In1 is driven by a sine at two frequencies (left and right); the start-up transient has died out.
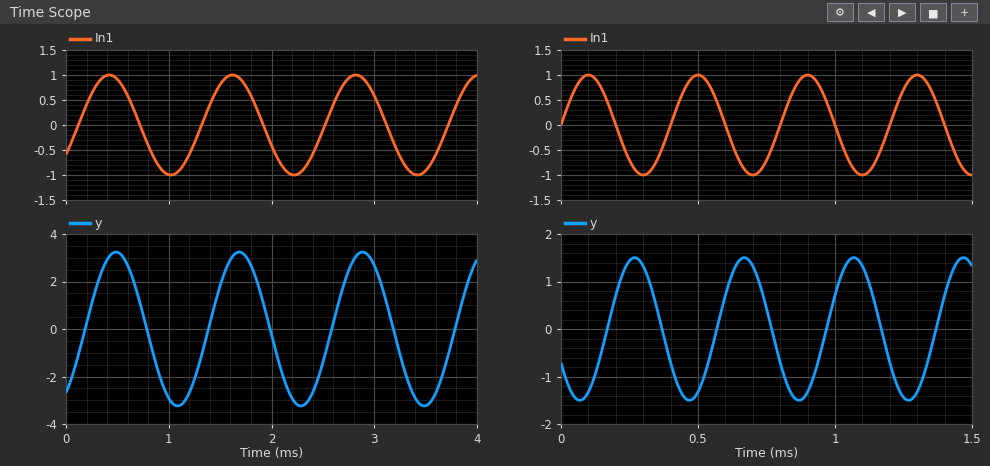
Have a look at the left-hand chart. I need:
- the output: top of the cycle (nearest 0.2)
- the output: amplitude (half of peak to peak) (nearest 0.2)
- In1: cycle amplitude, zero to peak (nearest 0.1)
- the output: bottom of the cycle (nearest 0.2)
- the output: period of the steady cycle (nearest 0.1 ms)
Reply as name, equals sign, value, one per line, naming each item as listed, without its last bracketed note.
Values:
the output: top of the cycle = 3.2
the output: amplitude (half of peak to peak) = 3.2
In1: cycle amplitude, zero to peak = 1.0
the output: bottom of the cycle = -3.2
the output: period of the steady cycle = 1.2 ms
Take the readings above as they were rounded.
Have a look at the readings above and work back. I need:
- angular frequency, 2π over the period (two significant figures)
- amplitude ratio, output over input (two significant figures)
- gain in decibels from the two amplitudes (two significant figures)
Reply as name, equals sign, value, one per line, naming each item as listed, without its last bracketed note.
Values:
angular frequency, 2π over the period = 5.2 rad/ms
amplitude ratio, output over input = 3.2
gain in decibels from the two amplitudes = 10 dB
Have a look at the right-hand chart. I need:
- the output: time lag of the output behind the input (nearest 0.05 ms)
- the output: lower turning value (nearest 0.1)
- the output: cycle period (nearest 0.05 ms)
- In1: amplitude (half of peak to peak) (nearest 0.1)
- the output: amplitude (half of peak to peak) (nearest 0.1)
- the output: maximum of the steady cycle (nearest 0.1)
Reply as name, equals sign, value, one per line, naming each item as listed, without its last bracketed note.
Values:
the output: time lag of the output behind the input = 0.15 ms
the output: lower turning value = -1.5
the output: cycle period = 0.40 ms
In1: amplitude (half of peak to peak) = 1.0
the output: amplitude (half of peak to peak) = 1.5
the output: maximum of the steady cycle = 1.5
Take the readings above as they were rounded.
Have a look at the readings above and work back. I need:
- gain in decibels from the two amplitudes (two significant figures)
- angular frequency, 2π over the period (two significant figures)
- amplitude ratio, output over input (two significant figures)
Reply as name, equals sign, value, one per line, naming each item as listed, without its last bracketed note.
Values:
gain in decibels from the two amplitudes = 3.5 dB
angular frequency, 2π over the period = 16 rad/ms
amplitude ratio, output over input = 1.5
